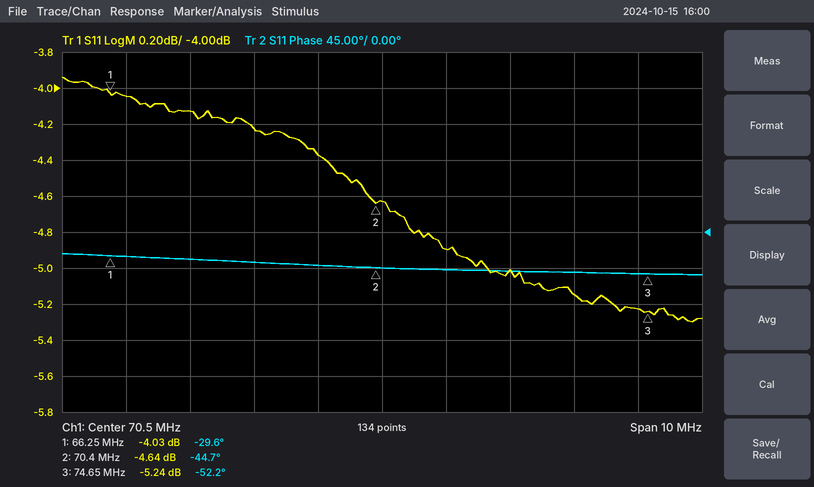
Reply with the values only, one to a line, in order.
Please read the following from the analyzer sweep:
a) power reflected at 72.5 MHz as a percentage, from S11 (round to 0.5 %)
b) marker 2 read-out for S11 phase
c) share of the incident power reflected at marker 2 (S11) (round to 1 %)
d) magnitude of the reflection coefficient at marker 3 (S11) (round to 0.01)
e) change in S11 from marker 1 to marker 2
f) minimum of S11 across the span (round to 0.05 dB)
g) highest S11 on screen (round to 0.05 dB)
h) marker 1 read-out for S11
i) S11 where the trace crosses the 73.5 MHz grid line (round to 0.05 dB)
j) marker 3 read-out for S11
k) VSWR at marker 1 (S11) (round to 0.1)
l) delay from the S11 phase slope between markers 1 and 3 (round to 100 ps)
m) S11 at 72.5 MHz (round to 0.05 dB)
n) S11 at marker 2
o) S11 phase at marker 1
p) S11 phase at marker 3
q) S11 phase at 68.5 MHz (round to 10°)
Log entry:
31.5 %
-44.7°
34 %
0.55
-0.61 dB
-5.30 dB
-3.95 dB
-4.03 dB
-5.15 dB
-5.24 dB
4.4
7.5 ns
-5.00 dB
-4.64 dB
-29.6°
-52.2°
-40°
